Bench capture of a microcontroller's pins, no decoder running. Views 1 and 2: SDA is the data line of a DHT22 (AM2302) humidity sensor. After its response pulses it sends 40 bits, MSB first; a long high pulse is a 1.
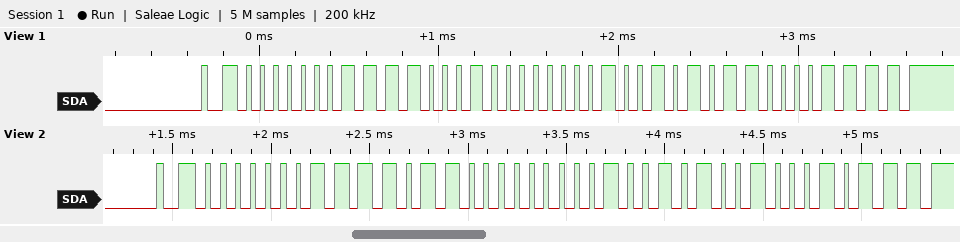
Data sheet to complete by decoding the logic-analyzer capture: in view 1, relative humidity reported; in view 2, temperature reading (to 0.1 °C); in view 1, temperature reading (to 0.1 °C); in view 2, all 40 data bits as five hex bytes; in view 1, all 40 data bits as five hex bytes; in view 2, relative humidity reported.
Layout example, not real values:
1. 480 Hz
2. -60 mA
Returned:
1. 48.2 %
2. 29.7 °C
3. 29.9 °C
4. 01 EC 01 29 17
5. 01 E2 01 2B 0F
6. 49.2 %
